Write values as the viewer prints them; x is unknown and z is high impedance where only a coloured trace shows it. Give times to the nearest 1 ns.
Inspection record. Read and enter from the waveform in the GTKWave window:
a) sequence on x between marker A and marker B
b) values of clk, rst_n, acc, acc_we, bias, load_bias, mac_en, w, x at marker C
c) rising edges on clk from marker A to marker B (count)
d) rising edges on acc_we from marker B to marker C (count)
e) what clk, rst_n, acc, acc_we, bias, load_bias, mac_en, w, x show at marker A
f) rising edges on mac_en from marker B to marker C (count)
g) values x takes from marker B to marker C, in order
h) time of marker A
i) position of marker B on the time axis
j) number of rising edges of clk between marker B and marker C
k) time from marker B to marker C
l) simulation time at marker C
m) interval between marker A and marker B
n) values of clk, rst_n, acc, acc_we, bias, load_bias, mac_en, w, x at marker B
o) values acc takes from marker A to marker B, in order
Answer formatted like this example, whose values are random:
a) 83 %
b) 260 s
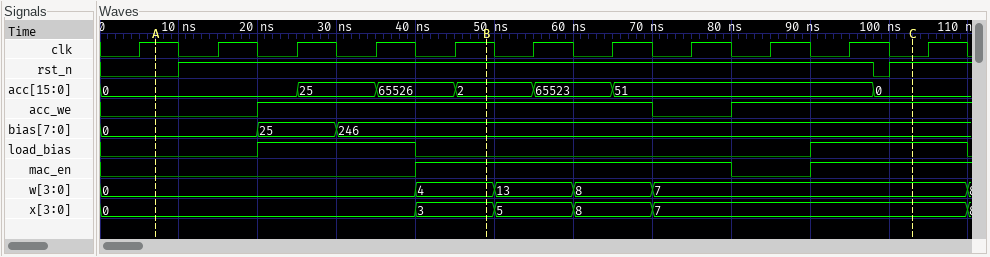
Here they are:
a) 0, 3
b) clk=0, rst_n=1, acc=0, acc_we=1, bias=246, load_bias=1, mac_en=1, w=7, x=7
c) 4
d) 1
e) clk=1, rst_n=0, acc=0, acc_we=0, bias=0, load_bias=0, mac_en=0, w=0, x=0
f) 1
g) 3, 5, 8, 7
h) 7 ns
i) 49 ns
j) 5
k) 54 ns
l) 103 ns
m) 42 ns
n) clk=1, rst_n=1, acc=2, acc_we=1, bias=246, load_bias=0, mac_en=1, w=4, x=3
o) 0, 25, 65526, 2
